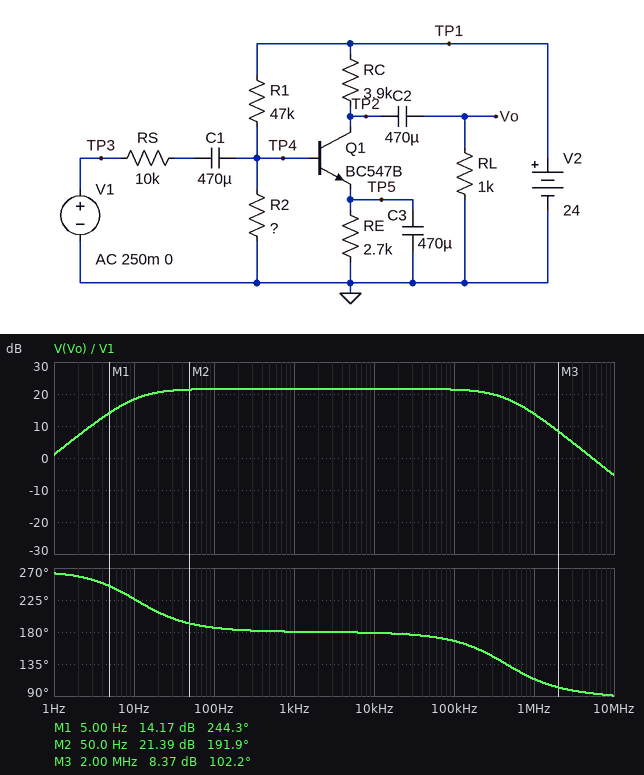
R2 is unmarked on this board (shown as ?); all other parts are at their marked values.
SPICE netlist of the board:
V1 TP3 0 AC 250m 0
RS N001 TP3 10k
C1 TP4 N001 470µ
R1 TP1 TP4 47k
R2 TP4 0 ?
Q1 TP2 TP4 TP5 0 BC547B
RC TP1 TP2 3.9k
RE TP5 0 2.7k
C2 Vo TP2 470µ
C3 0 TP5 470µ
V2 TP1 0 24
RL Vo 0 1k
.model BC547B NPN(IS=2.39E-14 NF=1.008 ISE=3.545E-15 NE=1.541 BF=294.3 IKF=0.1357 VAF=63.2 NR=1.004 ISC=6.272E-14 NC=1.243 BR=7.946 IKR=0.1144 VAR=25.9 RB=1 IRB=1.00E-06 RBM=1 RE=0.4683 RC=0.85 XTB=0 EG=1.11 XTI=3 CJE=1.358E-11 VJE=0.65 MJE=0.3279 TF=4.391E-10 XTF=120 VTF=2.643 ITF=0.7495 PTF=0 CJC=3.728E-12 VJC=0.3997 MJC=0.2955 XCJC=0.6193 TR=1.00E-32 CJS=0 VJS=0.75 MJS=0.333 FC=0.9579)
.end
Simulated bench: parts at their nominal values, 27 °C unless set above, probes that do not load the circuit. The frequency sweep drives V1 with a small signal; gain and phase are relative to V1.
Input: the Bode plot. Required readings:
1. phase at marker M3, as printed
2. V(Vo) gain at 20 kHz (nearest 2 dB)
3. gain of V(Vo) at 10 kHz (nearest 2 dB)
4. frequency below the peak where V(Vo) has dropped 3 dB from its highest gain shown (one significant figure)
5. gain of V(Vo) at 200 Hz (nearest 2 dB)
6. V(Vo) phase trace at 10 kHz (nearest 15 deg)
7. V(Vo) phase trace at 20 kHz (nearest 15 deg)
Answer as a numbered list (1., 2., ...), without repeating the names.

1. 102.2 deg
2. 22 dB
3. 22 dB
4. 10 Hz
5. 22 dB
6. 180 deg
7. 180 deg
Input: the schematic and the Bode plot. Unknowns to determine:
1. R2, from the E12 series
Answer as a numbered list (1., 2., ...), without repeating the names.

1. 12 kΩ
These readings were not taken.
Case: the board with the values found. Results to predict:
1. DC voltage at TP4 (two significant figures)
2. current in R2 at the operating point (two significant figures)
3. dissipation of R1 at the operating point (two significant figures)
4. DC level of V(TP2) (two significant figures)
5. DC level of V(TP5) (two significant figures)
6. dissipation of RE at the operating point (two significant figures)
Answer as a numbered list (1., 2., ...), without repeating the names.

1. 4.8 V
2. 400 µA
3. 7.8 mW
4. 18 V
5. 4.2 V
6. 6.5 mW
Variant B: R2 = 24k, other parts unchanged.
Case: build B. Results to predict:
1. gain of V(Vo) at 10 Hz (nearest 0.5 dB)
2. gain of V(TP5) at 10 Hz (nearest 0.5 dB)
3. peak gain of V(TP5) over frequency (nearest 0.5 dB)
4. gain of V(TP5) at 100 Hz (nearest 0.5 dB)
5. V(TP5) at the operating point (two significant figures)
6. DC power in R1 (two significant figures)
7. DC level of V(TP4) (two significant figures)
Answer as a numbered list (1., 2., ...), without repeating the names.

1. 20.5 dB
2. -7.0 dB
3. -4.5 dB
4. -23.5 dB
5. 7.3 V
6. 5.5 mW
7. 8.0 V
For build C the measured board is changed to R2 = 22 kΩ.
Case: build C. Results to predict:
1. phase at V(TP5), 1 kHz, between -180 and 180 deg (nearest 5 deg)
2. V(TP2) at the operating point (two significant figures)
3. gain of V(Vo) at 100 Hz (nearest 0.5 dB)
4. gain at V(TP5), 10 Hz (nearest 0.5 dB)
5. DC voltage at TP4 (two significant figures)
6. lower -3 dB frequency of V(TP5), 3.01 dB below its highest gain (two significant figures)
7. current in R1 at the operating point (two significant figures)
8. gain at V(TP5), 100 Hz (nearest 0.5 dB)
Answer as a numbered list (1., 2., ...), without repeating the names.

1. -90 deg
2. 14 V
3. 23.5 dB
4. -7.0 dB
5. 7.5 V
6. 14 mHz
7. 350 µA
8. -24.0 dB
